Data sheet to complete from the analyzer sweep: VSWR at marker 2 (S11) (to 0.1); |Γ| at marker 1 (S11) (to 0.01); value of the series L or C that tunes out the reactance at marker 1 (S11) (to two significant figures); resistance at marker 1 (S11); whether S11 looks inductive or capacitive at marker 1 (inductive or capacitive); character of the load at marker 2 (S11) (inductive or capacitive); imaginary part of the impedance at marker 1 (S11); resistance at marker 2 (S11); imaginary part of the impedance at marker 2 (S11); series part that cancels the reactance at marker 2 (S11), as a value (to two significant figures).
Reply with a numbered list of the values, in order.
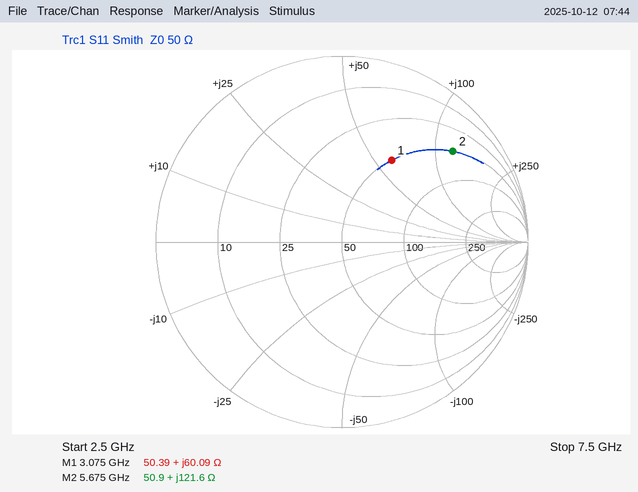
1. 7.7
2. 0.51
3. 860 fF
4. 50.39 Ω
5. inductive
6. inductive
7. +60.09 Ω
8. 50.9 Ω
9. +121.6 Ω
10. 230 fF
